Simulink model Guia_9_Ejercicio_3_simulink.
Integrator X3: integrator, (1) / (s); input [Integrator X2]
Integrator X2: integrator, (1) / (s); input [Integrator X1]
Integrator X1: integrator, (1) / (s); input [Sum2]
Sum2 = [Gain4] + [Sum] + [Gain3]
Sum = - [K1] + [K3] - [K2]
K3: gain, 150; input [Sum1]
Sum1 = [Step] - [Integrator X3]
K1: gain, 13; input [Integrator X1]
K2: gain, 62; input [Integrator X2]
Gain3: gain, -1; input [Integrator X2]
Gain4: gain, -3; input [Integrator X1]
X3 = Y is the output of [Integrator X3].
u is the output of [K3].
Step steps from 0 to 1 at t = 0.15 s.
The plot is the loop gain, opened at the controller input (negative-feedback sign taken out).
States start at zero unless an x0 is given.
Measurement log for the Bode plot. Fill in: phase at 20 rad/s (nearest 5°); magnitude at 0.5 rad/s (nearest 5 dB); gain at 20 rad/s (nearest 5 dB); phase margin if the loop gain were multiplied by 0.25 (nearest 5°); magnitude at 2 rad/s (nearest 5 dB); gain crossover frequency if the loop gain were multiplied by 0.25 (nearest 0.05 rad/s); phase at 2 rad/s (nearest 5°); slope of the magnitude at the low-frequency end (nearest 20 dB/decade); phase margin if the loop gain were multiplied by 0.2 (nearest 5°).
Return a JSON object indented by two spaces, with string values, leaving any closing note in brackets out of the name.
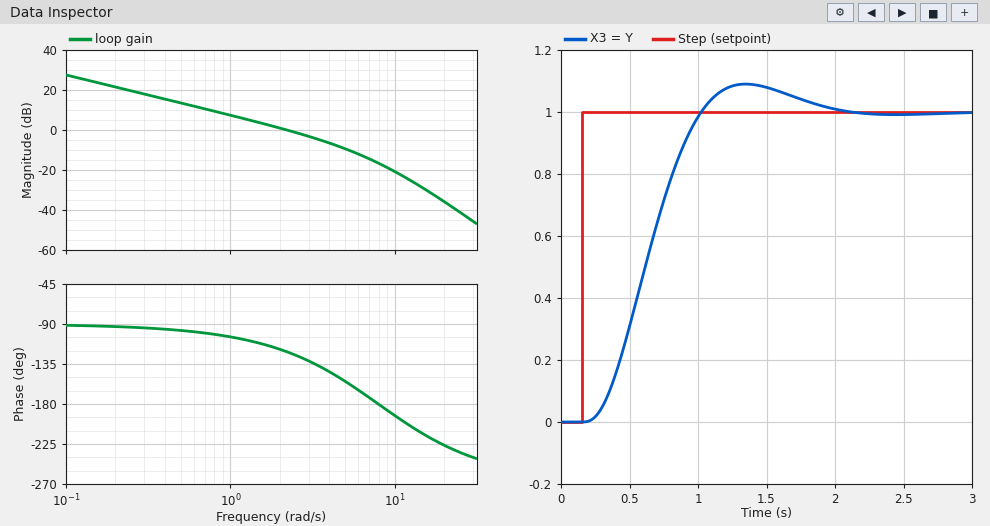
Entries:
{
  "phase at 20 rad/s": "-225°",
  "magnitude at 0.5 rad/s": "15 dB",
  "gain at 20 rad/s": "-35 dB",
  "phase margin if the loop gain were multiplied by 0.25": "80°",
  "magnitude at 2 rad/s": "0 dB",
  "gain crossover frequency if the loop gain were multiplied by 0.25": "0.60 rad/s",
  "phase at 2 rad/s": "-120°",
  "slope of the magnitude at the low-frequency end": "-20 dB/decade",
  "phase margin if the loop gain were multiplied by 0.2": "85°"
}
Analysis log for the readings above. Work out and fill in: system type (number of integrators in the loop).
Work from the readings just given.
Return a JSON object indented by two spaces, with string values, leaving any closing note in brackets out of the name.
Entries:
{
  "system type": "1"
}
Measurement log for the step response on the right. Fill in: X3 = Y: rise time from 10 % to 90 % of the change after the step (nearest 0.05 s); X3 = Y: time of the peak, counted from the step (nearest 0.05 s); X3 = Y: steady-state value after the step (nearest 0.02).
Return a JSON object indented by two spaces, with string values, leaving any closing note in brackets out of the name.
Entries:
{
  "X3 = Y: rise time from 10 % to 90 % of the change after the step": "0.55 s",
  "X3 = Y: time of the peak, counted from the step": "1.20 s",
  "X3 = Y: steady-state value after the step": "1.00"
}
